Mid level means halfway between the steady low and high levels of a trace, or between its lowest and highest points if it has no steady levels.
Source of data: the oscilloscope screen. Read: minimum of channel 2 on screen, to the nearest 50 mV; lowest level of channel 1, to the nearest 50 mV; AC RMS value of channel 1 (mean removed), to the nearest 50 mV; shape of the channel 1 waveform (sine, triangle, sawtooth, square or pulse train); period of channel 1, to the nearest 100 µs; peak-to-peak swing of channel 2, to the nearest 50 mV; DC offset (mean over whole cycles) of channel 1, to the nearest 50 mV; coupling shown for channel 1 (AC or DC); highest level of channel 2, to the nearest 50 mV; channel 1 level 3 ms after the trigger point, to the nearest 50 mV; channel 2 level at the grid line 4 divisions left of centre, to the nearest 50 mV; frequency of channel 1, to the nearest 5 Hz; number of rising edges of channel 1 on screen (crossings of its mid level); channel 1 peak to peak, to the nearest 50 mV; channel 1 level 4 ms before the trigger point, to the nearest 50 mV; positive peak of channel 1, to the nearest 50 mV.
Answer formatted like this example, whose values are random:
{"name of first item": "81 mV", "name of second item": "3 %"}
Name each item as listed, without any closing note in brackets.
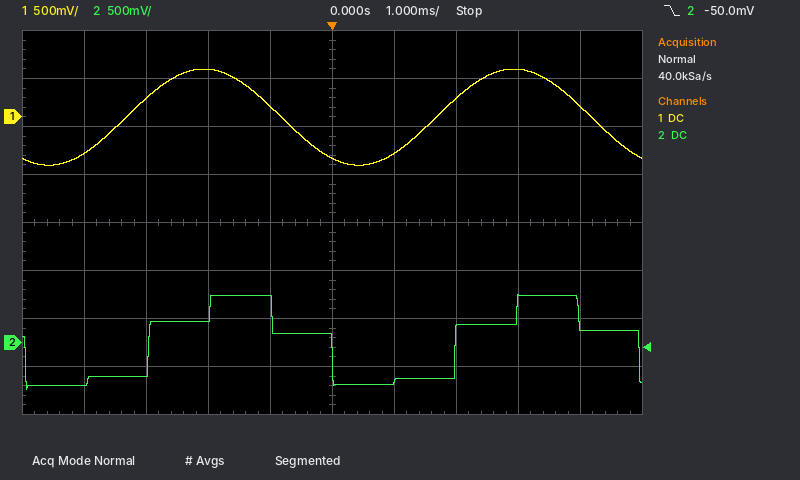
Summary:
{"minimum of channel 2 on screen, to the nearest 50 mV": "-500 mV", "lowest level of channel 1, to the nearest 50 mV": "-500 mV", "AC RMS value of channel 1 (mean removed), to the nearest 50 mV": "350 mV", "shape of the channel 1 waveform": "sine", "period of channel 1, to the nearest 100 µs": "5.0 ms", "peak-to-peak swing of channel 2, to the nearest 50 mV": "1.00 V", "DC offset (mean over whole cycles) of channel 1, to the nearest 50 mV": "0 mV", "coupling shown for channel 1": "DC", "highest level of channel 2, to the nearest 50 mV": "500 mV", "channel 1 level 3 ms after the trigger point, to the nearest 50 mV": "500 mV", "channel 2 level at the grid line 4 divisions left of centre, to the nearest 50 mV": "-450 mV", "frequency of channel 1, to the nearest 5 Hz": "200 Hz", "number of rising edges of channel 1 on screen": "2", "channel 1 peak to peak, to the nearest 50 mV": "1.00 V", "channel 1 level 4 ms before the trigger point, to the nearest 50 mV": "-400 mV", "positive peak of channel 1, to the nearest 50 mV": "500 mV"}
